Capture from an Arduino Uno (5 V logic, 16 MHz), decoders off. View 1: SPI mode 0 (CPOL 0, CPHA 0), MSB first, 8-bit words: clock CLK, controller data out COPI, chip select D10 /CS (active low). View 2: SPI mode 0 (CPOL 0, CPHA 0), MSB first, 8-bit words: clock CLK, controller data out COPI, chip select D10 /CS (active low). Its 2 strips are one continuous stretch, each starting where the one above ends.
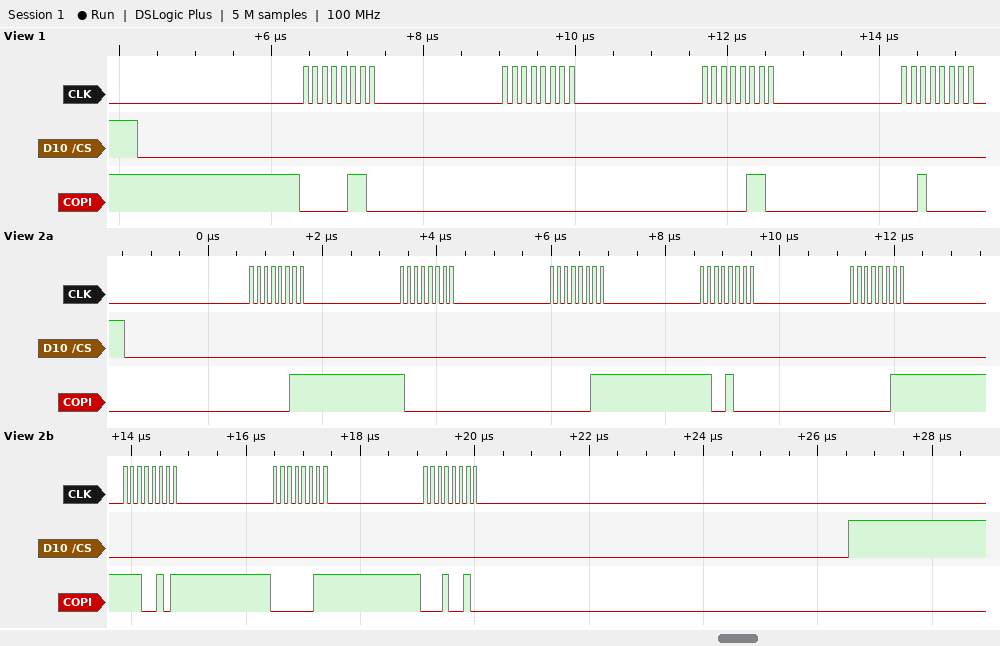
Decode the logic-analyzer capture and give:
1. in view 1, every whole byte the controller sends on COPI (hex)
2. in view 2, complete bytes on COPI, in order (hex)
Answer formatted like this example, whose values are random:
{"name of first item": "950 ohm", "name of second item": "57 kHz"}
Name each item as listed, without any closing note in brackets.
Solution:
{"in view 1, every whole byte the controller sends on COPI": "06 00 06 20", "in view 2, complete bytes on COPI, in order": "03 80 03 C8 03 E5 03 12"}
